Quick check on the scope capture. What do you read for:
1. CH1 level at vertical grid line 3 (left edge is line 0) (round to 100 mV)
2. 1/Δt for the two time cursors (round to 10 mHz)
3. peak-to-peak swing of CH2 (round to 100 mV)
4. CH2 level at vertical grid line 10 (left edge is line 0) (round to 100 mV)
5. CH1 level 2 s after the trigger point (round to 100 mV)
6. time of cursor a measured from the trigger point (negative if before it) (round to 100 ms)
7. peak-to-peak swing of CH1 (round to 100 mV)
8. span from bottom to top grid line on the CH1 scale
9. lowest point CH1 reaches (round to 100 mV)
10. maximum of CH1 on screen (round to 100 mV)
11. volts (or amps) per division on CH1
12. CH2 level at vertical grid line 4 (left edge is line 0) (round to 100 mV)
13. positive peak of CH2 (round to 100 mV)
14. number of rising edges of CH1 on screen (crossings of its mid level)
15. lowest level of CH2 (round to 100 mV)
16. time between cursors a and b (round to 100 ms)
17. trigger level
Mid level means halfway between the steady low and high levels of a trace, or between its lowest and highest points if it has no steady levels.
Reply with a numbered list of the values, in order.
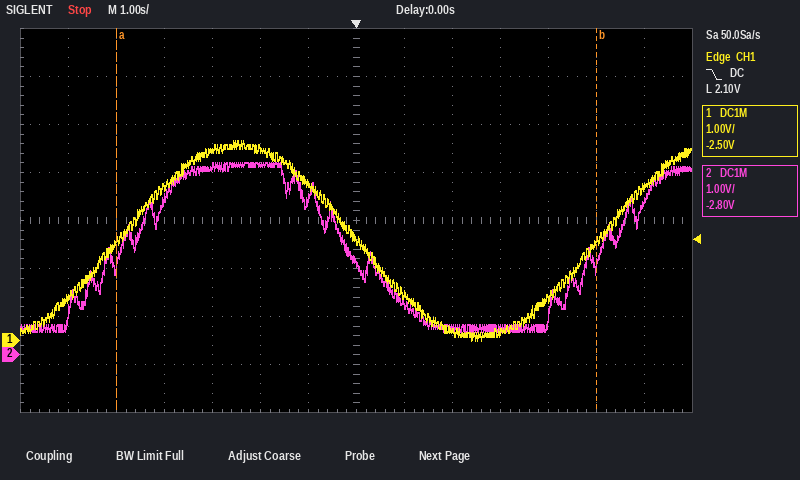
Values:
1. 3.2 V
2. 100 mHz
3. 3.5 V
4. 600 mV
5. 200 mV
6. -5.0 s
7. 4.2 V
8. 8 V
9. 0.0 V
10. 4.2 V
11. 1 V
12. 3.9 V
13. 4.0 V
14. 2
15. 500 mV
16. 10.0 s
17. 2.10 V
